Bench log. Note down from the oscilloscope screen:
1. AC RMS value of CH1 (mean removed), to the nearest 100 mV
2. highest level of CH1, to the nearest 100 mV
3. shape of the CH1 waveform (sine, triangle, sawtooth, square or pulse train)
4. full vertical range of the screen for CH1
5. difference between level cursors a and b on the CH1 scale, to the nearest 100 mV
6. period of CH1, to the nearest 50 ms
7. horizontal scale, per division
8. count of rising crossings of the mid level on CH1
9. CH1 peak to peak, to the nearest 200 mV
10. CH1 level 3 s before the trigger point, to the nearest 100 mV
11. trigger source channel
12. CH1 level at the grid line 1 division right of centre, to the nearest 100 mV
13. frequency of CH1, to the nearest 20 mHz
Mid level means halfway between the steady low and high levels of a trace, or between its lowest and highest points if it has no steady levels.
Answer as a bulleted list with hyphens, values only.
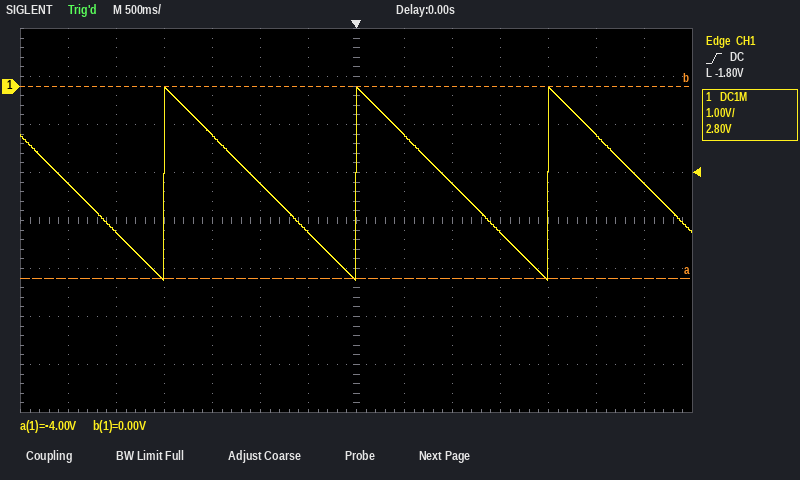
- 1.2 V
- 0.0 V
- sawtooth
- 8 V
- 4.0 V
- 2.00 s
- 500 ms
- 3
- 4.0 V
- -2.0 V
- CH1
- -1.0 V
- 500 mHz
